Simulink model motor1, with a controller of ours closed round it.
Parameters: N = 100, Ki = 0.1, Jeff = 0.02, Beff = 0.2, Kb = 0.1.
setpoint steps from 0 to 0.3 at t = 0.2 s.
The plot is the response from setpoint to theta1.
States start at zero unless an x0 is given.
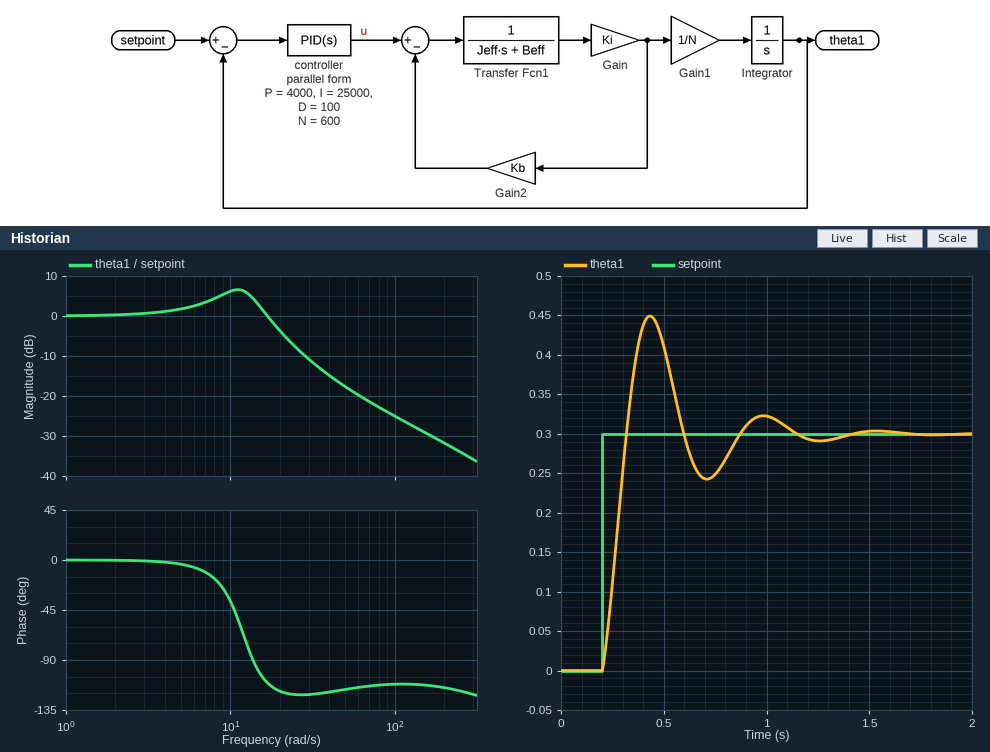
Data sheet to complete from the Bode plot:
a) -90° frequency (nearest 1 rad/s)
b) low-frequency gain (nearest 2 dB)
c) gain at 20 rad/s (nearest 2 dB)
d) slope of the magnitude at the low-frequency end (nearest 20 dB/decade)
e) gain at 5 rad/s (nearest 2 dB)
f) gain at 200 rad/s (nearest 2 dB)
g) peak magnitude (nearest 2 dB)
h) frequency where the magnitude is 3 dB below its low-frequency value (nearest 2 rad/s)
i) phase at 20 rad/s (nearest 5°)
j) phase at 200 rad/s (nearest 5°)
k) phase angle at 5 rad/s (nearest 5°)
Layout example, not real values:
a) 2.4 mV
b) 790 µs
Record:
a) 14 rad/s
b) 0 dB
c) -4 dB
d) 0 dB/decade
e) 2 dB
f) -32 dB
g) 6 dB
h) 20 rad/s
i) -120°
j) -115°
k) -5°
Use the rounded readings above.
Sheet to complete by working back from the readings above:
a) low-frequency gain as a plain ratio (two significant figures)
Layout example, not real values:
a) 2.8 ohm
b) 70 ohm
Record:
a) 1.0
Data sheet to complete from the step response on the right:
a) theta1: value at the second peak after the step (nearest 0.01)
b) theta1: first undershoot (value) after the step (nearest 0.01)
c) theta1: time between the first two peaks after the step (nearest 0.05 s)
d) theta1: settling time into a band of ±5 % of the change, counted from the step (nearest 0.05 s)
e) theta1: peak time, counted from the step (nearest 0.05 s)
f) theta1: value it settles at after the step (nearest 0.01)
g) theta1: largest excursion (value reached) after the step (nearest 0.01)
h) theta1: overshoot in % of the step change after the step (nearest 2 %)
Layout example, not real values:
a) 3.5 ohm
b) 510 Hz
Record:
a) 0.32
b) 0.24
c) 0.55 s
d) 0.85 s
e) 0.25 s
f) 0.30
g) 0.45
h) 50 %
